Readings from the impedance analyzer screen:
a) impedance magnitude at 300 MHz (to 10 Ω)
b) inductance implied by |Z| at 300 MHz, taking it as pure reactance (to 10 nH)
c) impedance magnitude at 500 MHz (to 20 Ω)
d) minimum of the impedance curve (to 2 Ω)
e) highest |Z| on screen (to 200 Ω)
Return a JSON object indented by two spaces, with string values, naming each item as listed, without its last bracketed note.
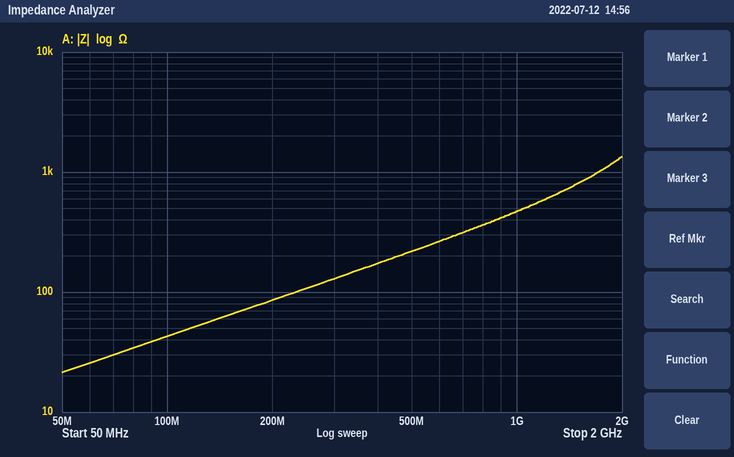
{
  "impedance magnitude at 300 MHz": "130 Ω",
  "inductance implied by |Z| at 300 MHz, taking it as pure reactance": "70 nH",
  "impedance magnitude at 500 MHz": "220 Ω",
  "minimum of the impedance curve": "22 Ω",
  "highest |Z| on screen": "1.4 kΩ"
}
